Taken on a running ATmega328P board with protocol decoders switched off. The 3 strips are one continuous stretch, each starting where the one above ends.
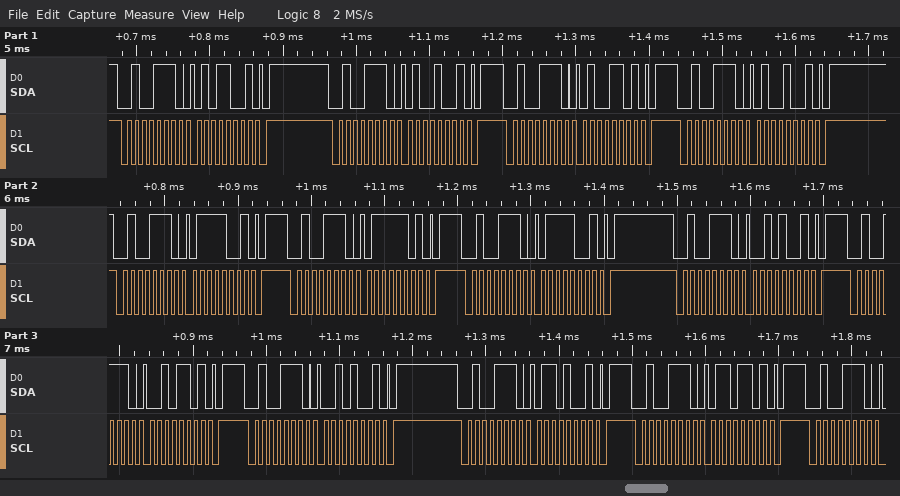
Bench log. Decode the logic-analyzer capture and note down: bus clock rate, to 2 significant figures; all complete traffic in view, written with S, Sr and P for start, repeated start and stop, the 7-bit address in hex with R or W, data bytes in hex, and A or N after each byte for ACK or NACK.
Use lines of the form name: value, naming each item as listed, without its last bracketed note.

bus clock rate, to 2 significant figures: 100 kHz
all complete traffic in view, written with S, Sr and P for start, repeated start and stop, the 7-bit address in hex with R or W, data bytes in hex, and A or N after each byte for ACK or NACK: S 27W A 59 A P S 27W A 49 A P S 27W A 4D A P S 27W A 49 A P S 27W A 79 A P S 27W A 7D A P S 27W A 79 A P S 27W A 29 A P S 27W A 2D A P S 27W A 29 A P S 27W A 69 A P S 27W A 6D A P S 27W A
